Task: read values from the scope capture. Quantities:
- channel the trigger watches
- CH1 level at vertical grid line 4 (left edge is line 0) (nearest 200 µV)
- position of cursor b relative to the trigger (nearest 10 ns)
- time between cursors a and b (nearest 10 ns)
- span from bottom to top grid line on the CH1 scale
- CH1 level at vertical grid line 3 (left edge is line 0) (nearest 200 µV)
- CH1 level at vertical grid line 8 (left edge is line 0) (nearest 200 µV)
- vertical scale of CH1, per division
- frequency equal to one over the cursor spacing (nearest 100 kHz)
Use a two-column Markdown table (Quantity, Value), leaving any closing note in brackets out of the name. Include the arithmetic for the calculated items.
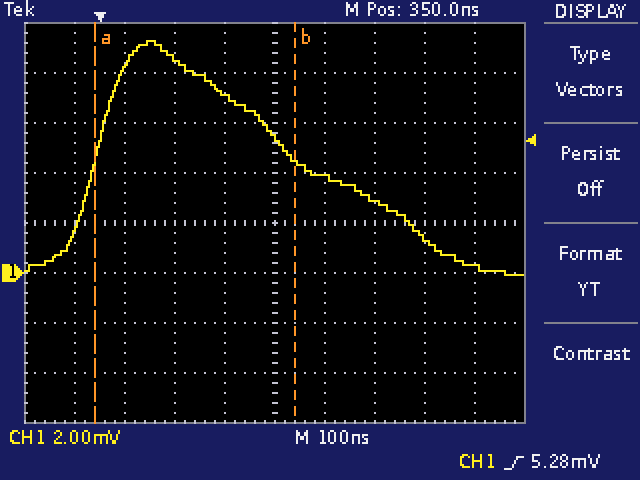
| Quantity | Value |
|---|---|
| channel the trigger watches | CH1 |
| CH1 level at vertical grid line 4 (left edge is line 0) | 7.2 mV |
| position of cursor b relative to the trigger | +390 ns |
| time between cursors a and b | 400 ns |
| span from bottom to top grid line on the CH1 scale | 16 mV |
| CH1 level at vertical grid line 3 (left edge is line 0) | 8.6 mV |
| CH1 level at vertical grid line 8 (left edge is line 0) | 1.4 mV |
| vertical scale of CH1, per division | 2 mV |
| frequency equal to one over the cursor spacing | 1 / 400 ns ≈ 2.5 MHz |
